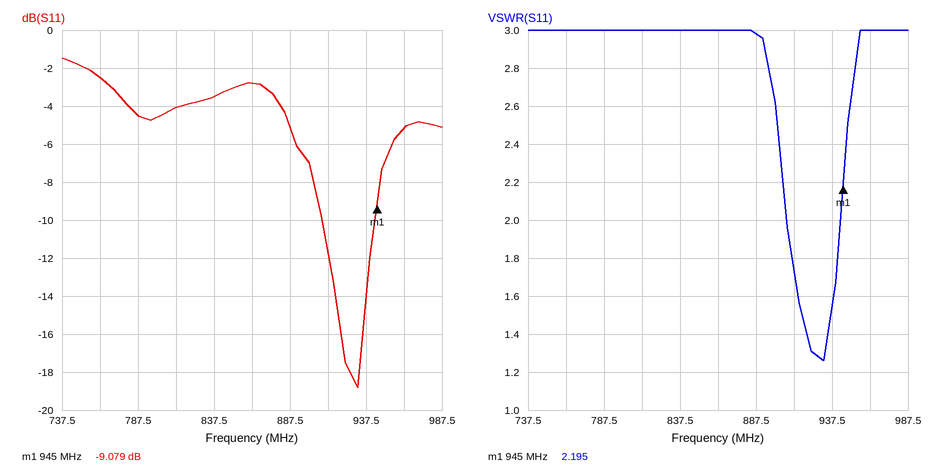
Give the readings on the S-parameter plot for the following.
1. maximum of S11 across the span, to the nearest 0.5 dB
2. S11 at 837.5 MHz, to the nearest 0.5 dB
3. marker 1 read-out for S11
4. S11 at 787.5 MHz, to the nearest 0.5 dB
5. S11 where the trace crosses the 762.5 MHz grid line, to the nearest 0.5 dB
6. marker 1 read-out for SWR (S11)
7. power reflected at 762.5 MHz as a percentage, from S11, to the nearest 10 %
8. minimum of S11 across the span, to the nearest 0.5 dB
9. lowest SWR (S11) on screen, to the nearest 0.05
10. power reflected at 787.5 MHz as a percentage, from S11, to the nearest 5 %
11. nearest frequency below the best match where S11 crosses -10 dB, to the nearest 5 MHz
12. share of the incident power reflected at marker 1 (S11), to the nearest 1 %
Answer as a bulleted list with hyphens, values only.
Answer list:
- -1.5 dB
- -3.5 dB
- -9.079 dB
- -4.5 dB
- -2.5 dB
- 2.195
- 60 %
- -19.0 dB
- 1.25
- 35 %
- 910 MHz
- 12 %
